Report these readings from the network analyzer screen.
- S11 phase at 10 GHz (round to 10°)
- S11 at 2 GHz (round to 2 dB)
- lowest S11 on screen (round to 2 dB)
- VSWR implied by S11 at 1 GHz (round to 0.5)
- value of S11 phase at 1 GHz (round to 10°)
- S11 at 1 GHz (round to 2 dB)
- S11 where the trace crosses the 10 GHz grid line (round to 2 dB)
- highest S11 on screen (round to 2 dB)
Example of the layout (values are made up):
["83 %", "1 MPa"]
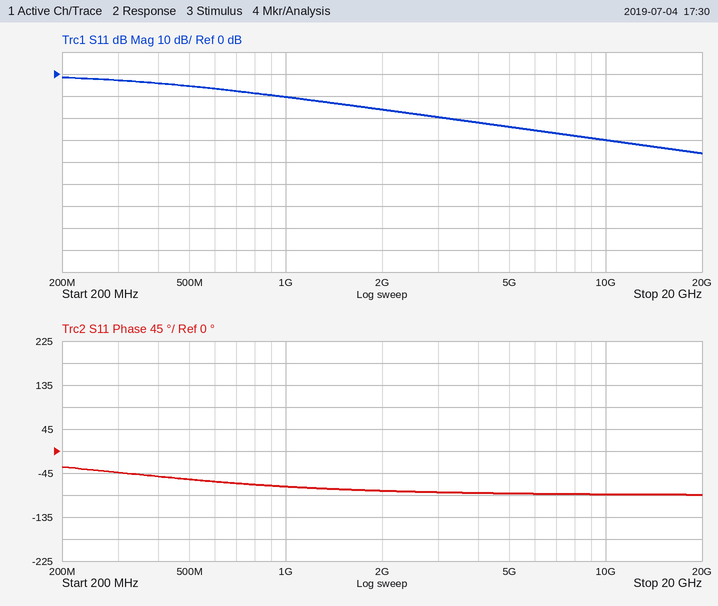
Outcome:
["-90°", "-16 dB", "-36 dB", "2.0", "-70°", "-10 dB", "-30 dB", "-2 dB"]
